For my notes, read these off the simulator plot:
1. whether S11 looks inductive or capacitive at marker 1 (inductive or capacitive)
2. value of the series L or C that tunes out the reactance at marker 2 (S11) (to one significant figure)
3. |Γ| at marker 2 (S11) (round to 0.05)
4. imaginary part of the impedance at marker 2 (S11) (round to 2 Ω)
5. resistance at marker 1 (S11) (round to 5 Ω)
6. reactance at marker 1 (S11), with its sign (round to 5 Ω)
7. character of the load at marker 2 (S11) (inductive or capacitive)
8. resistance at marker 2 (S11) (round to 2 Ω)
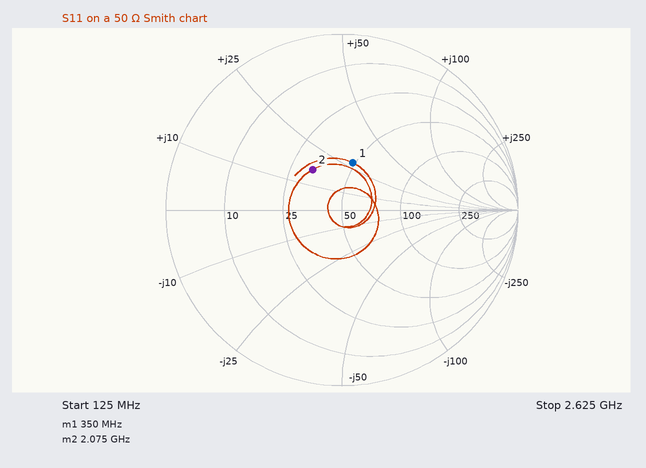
inductive
5 pF
0.30
+16 Ω
50 Ω
+30 Ω
inductive
32 Ω
